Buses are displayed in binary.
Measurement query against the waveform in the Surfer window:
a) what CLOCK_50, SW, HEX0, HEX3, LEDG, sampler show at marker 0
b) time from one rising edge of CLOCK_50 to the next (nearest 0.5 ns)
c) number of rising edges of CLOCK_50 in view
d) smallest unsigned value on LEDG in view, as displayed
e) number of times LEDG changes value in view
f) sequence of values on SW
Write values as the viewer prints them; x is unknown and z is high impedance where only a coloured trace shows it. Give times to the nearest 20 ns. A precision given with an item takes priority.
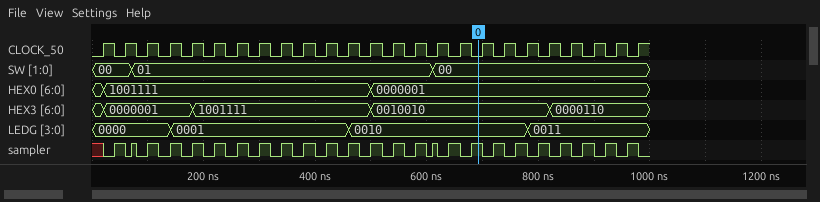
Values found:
CLOCK_50=0, SW=00, HEX0=0000001, HEX3=0010010, LEDG=0010, sampler=1
40 ns
25
0000
3
00, 01, 00
